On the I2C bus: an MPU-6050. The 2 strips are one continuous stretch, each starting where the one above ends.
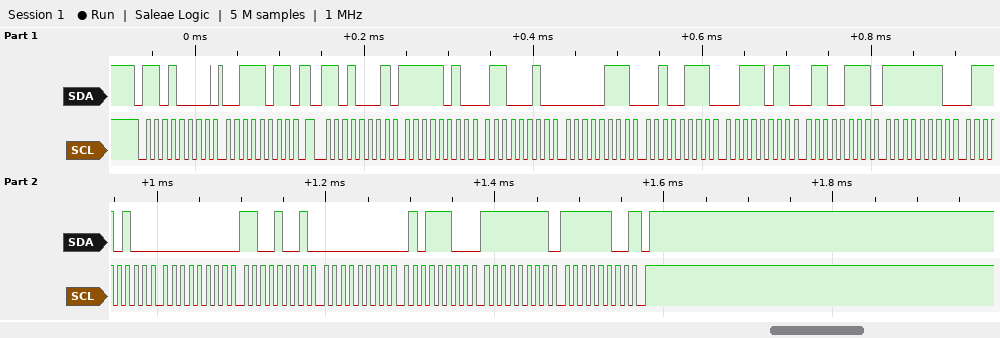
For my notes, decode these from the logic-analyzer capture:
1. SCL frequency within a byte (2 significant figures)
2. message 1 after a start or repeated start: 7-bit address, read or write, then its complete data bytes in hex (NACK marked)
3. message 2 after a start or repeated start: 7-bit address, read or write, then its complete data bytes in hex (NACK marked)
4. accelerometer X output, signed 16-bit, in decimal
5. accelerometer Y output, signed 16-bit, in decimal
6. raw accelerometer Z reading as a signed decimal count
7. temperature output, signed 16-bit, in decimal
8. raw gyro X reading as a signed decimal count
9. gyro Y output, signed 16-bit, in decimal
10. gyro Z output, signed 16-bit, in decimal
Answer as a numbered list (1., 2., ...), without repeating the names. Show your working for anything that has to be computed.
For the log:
1. 100 kHz
2. 0x68 write: 3B
3. 0x68 read: FA 62 07 27 3B 67 FE 74 00 C9 00 5C FF FC NACK
4. 0xFA62 = -1438
5. 0x0727 = 1831
6. 0x3B67 = 15207
7. 0xFE74 = -396
8. 0x00C9 = 201
9. 0x005C = 92
10. 0xFFFC = -4
